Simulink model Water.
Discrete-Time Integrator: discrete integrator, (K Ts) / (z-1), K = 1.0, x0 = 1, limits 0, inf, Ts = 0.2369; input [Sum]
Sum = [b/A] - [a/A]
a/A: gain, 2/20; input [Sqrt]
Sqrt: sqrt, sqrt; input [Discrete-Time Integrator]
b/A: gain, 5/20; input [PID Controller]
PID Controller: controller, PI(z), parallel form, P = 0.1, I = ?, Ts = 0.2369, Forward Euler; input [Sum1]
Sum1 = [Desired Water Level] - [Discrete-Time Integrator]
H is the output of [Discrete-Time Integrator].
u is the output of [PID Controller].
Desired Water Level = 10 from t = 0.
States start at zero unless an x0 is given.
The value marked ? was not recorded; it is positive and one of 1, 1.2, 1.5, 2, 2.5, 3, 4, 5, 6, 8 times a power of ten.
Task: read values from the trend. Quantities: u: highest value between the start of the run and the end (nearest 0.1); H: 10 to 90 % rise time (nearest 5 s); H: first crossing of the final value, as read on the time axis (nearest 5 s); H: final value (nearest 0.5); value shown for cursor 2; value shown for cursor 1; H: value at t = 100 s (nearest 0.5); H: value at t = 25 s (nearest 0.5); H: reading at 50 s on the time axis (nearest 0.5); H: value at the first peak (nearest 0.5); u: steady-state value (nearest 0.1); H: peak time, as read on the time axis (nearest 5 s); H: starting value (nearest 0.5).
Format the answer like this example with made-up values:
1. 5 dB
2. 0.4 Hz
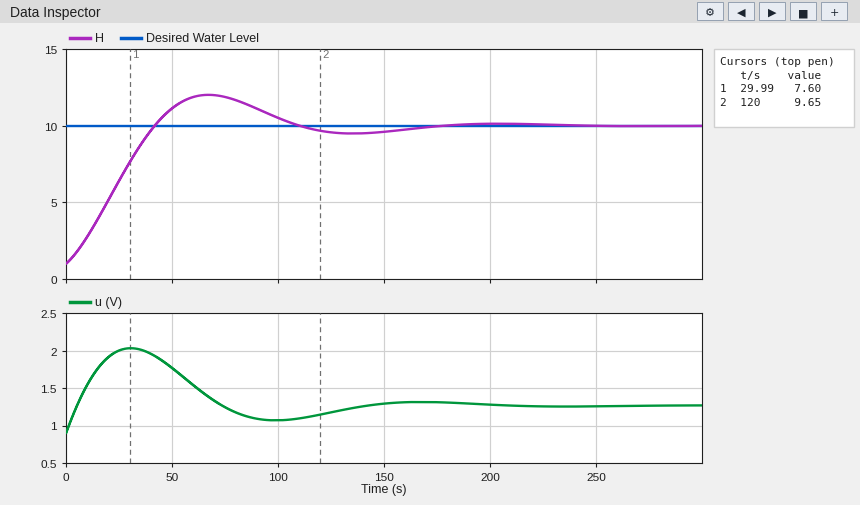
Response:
1. 2.0
2. 30 s
3. 40 s
4. 10.0
5. 9.65
6. 7.60
7. 10.5
8. 6.5
9. 11.0
10. 12.0
11. 1.3
12. 65 s
13. 1.0
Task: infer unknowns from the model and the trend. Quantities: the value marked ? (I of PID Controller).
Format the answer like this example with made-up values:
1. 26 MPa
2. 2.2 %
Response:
1. 0.01
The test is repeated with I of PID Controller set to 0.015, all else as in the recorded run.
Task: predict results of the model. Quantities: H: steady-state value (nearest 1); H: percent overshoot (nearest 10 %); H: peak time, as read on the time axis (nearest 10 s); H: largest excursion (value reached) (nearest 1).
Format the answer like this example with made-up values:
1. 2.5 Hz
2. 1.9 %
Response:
1. 10
2. 30 %
3. 50 s
4. 13
